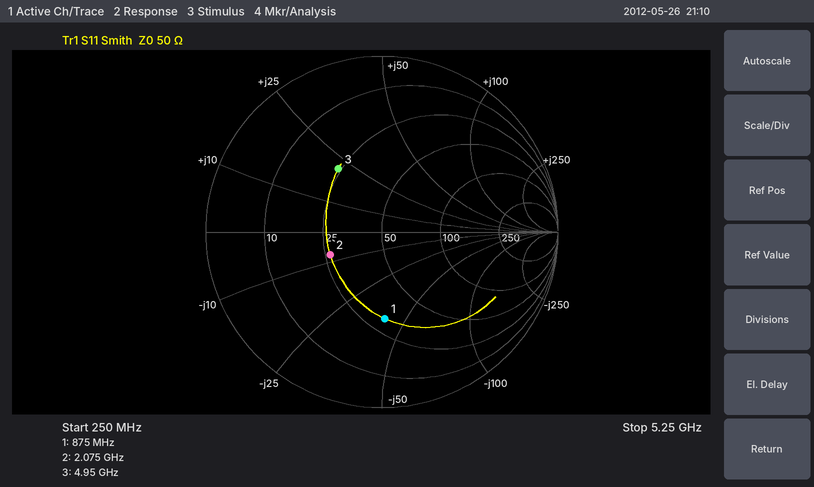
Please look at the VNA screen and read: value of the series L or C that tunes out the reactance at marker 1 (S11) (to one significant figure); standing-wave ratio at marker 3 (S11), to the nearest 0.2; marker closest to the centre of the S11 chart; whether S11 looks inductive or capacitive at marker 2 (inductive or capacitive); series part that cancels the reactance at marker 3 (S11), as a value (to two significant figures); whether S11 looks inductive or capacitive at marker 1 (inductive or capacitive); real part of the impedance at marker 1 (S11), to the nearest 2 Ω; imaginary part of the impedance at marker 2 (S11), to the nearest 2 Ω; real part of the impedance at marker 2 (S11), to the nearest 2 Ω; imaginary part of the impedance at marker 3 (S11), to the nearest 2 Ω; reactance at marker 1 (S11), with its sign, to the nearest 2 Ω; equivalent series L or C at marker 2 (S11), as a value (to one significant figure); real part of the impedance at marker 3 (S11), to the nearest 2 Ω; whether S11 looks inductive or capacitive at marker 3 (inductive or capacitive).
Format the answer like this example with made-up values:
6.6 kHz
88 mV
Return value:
7 nH
2.6
marker 2
capacitive
1.5 pF
capacitive
32 Ω
-8 Ω
26 Ω
+22 Ω
-40 Ω
10 pF
24 Ω
inductive
